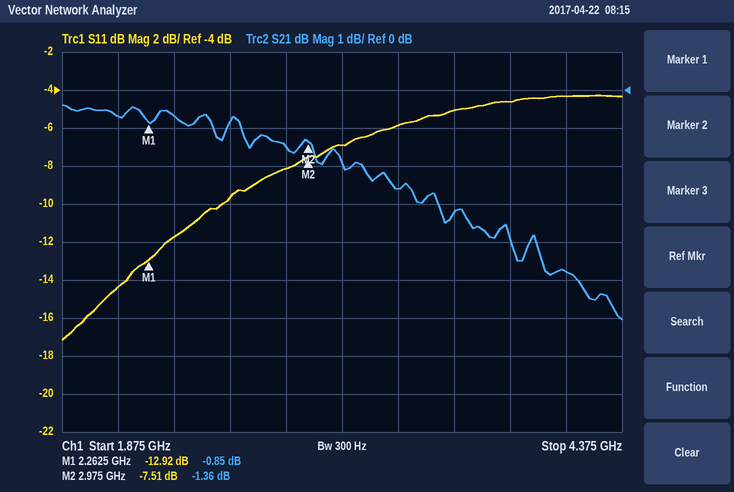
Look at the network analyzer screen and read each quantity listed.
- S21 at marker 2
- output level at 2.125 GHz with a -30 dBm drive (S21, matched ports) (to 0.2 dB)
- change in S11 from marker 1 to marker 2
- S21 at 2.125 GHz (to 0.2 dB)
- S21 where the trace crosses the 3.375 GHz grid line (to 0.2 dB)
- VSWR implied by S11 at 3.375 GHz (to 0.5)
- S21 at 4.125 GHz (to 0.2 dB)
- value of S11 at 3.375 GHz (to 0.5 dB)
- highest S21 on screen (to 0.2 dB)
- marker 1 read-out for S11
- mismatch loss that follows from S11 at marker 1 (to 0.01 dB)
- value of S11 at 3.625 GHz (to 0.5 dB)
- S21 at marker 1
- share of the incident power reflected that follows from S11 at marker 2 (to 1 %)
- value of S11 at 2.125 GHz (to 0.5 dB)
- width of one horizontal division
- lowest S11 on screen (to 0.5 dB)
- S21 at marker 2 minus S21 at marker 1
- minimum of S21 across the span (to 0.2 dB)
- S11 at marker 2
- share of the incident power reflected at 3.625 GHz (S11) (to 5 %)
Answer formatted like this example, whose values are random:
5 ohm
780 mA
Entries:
-1.36 dB
-30.6 dBm
5.41 dB
-0.6 dB
-2.6 dB
3.0
-4.8 dB
-6.0 dB
-0.4 dB
-12.92 dB
0.23 dB
-5.0 dB
-0.85 dB
18 %
-14.5 dB
250 MHz
-17.0 dB
-0.51 dB
-6.0 dB
-7.51 dB
30 %
